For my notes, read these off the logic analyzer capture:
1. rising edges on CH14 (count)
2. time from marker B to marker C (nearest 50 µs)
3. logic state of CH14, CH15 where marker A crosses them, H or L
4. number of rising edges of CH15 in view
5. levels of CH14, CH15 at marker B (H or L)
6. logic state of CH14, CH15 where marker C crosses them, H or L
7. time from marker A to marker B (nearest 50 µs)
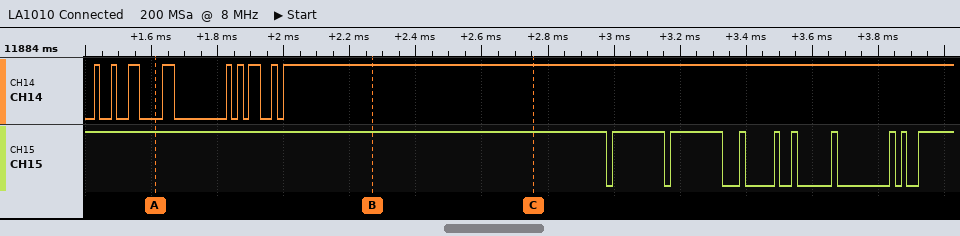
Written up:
9
500 µs
CH14=L, CH15=H
9
CH14=H, CH15=H
CH14=H, CH15=H
650 µs
